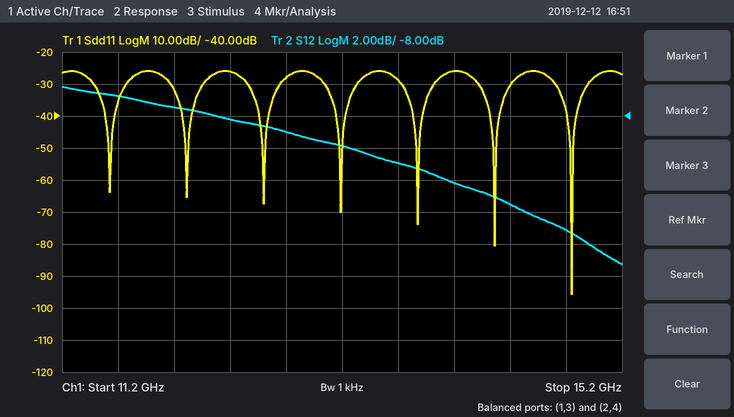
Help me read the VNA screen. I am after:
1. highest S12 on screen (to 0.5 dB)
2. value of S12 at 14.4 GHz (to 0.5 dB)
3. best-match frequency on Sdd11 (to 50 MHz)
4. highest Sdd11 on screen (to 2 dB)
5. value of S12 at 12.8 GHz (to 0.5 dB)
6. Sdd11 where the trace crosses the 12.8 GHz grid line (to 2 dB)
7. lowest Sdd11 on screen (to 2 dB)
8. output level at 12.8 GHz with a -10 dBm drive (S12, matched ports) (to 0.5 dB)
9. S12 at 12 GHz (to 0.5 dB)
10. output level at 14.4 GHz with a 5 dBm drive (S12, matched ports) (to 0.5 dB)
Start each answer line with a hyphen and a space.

- -6.0 dB
- -13.5 dB
- 14.85 GHz
- -26 dB
- -9.0 dB
- -28 dB
- -96 dB
- -19.0 dBm
- -7.5 dB
- -8.5 dBm
